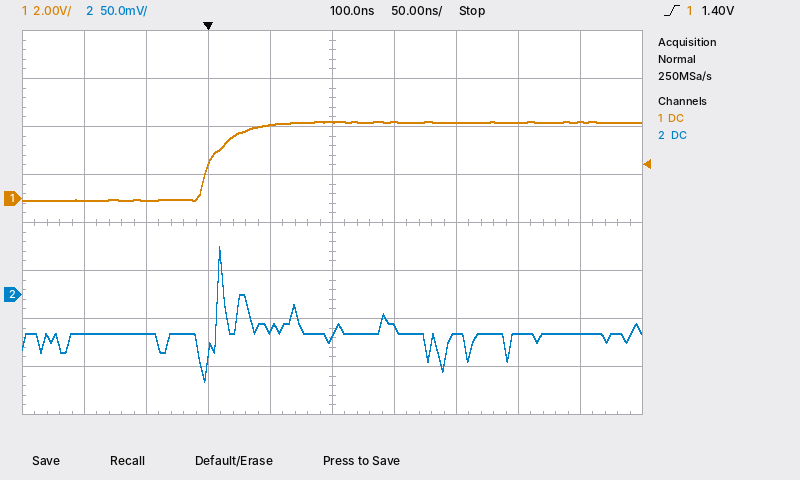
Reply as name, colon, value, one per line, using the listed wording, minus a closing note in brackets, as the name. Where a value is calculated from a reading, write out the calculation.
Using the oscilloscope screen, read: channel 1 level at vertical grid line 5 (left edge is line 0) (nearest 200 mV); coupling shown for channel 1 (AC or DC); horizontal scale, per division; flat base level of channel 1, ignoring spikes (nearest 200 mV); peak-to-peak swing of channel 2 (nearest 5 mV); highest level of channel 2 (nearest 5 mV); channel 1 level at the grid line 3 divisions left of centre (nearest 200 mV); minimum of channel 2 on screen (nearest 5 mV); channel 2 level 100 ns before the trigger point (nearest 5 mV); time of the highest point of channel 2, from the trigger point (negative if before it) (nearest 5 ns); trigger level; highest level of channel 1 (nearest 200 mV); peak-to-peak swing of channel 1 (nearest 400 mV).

channel 1 level at vertical grid line 5 (left edge is line 0): 3.2 V
coupling shown for channel 1: DC
horizontal scale, per division: 50 ns
flat base level of channel 1, ignoring spikes: 0.0 V
peak-to-peak swing of channel 2: 50 mV − (-90 mV) = 140 mV
highest level of channel 2: 50 mV
channel 1 level at the grid line 3 divisions left of centre: 0.0 V
minimum of channel 2 on screen: -90 mV
channel 2 level 100 ns before the trigger point: -40 mV
time of the highest point of channel 2, from the trigger point (negative if before it): +10 ns
trigger level: 1.40 V
highest level of channel 1: 3.2 V
peak-to-peak swing of channel 1: 3.2 V
